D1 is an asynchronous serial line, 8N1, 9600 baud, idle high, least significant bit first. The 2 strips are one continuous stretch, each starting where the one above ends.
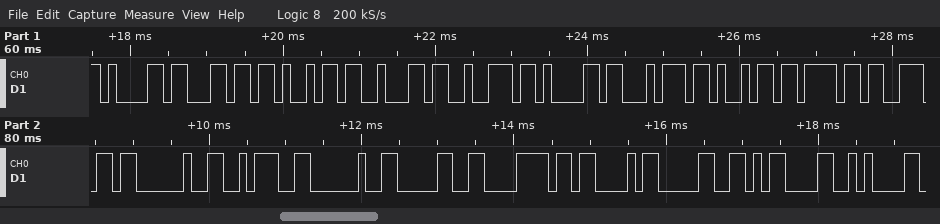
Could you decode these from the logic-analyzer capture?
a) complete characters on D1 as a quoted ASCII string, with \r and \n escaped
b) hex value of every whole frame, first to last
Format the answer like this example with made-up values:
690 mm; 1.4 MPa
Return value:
"alibration : 0xC0\r\n"; 61 6C 69 62 72 61 74 69 6F 6E 20 3A 20 30 78 43 30 0D 0A
